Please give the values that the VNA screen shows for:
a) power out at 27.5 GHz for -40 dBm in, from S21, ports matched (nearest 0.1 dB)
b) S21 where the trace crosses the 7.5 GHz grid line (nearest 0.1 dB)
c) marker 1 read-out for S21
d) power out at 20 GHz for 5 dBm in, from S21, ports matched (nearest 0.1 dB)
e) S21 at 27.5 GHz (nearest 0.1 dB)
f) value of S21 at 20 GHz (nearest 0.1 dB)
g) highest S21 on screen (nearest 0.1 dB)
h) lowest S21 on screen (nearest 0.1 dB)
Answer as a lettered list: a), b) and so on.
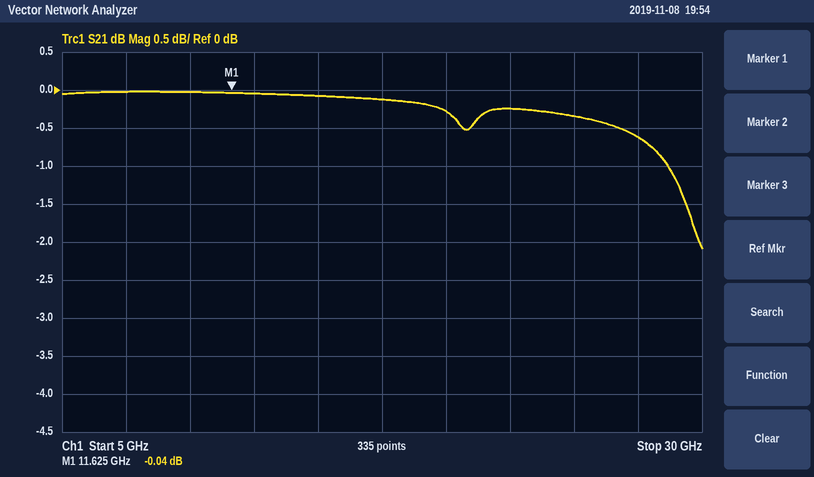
a) -40.6 dBm
b) 0.0 dB
c) -0.04 dB
d) 4.7 dBm
e) -0.6 dB
f) -0.3 dB
g) 0.0 dB
h) -2.1 dB
